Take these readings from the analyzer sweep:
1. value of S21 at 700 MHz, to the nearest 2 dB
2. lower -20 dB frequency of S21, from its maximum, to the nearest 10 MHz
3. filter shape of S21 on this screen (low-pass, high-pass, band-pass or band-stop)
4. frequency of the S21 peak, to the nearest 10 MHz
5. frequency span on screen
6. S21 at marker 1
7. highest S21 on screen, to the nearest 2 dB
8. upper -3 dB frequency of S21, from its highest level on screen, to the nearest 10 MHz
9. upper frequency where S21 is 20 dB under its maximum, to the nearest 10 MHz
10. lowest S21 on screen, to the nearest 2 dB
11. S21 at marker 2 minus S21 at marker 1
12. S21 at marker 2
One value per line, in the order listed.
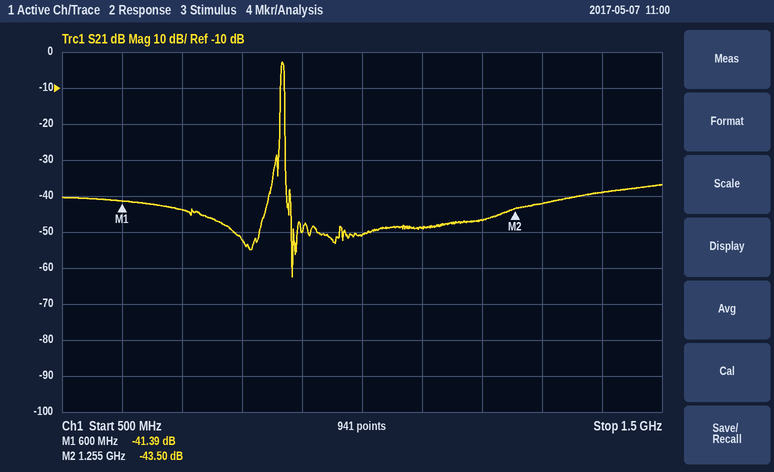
-44 dB
860 MHz
band-pass
870 MHz
1 GHz
-41.39 dB
-2 dB
870 MHz
870 MHz
-62 dB
-2.11 dB
-43.50 dB
